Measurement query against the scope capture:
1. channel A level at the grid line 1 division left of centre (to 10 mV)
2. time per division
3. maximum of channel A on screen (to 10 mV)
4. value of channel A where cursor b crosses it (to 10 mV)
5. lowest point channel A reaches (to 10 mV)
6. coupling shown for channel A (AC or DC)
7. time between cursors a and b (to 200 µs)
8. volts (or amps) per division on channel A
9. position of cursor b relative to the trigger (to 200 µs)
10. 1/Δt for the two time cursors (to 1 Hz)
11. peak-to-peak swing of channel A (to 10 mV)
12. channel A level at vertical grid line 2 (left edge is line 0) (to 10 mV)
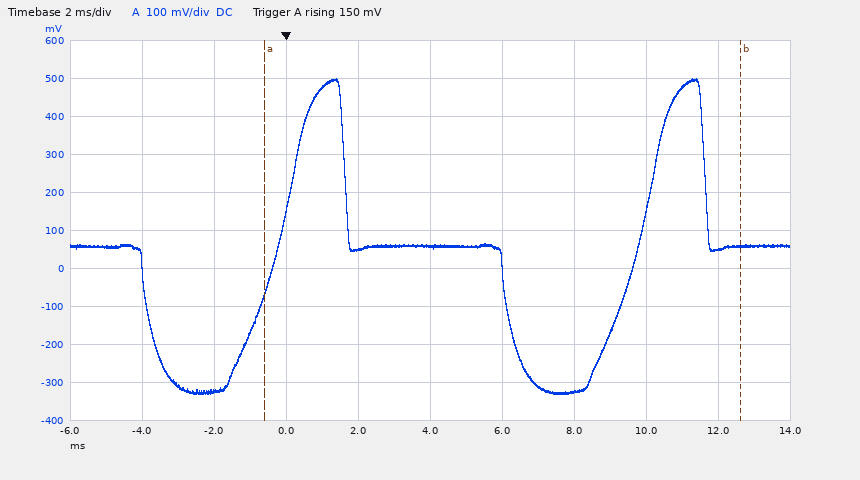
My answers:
50 mV
2 ms
500 mV
60 mV
-330 mV
DC
13.2 ms
100 mV
+12.6 ms
76 Hz
830 mV
-320 mV
